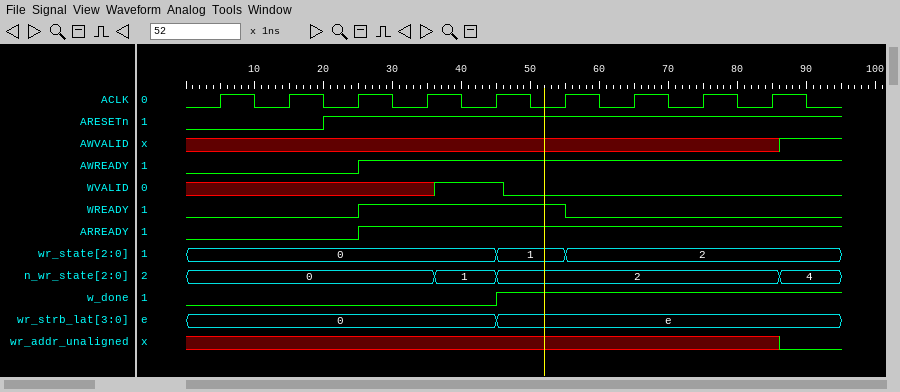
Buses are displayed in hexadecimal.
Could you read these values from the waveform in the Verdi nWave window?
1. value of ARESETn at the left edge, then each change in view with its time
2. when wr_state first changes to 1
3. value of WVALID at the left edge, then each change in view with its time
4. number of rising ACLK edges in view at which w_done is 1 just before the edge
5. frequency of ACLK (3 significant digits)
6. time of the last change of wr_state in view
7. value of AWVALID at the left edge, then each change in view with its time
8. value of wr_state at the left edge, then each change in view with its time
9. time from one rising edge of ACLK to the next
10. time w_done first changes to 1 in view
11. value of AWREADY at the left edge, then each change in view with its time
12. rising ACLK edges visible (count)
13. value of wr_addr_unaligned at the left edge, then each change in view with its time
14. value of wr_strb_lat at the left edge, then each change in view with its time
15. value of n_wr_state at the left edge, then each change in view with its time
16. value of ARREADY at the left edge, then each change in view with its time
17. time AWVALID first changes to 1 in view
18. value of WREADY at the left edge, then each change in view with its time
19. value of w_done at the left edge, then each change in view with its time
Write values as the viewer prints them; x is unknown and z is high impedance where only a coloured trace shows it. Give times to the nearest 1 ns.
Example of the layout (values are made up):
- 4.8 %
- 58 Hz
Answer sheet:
- 0, 1 at 20 ns
- 45 ns
- x, 1 at 36 ns, 0 at 46 ns
- 4
- 100 MHz
- 55 ns
- x, 1 at 86 ns
- 0, 1 at 45 ns, 2 at 55 ns
- 10 ns
- 45 ns
- 0, 1 at 25 ns
- 9
- x, 0 at 86 ns
- 0, e at 45 ns
- 0, 1 at 36 ns, 2 at 45 ns, 4 at 86 ns
- 0, 1 at 25 ns
- 86 ns
- 0, 1 at 25 ns, 0 at 55 ns
- 0, 1 at 45 ns
